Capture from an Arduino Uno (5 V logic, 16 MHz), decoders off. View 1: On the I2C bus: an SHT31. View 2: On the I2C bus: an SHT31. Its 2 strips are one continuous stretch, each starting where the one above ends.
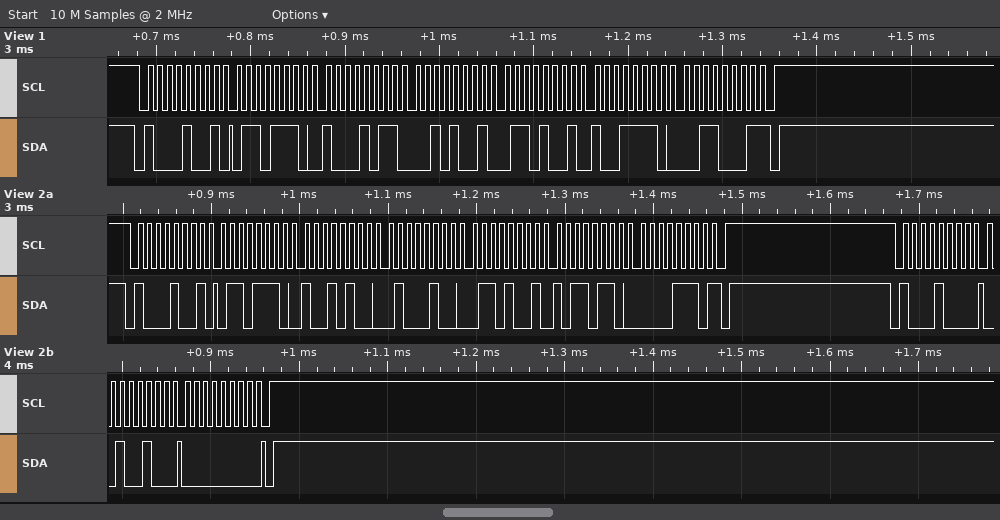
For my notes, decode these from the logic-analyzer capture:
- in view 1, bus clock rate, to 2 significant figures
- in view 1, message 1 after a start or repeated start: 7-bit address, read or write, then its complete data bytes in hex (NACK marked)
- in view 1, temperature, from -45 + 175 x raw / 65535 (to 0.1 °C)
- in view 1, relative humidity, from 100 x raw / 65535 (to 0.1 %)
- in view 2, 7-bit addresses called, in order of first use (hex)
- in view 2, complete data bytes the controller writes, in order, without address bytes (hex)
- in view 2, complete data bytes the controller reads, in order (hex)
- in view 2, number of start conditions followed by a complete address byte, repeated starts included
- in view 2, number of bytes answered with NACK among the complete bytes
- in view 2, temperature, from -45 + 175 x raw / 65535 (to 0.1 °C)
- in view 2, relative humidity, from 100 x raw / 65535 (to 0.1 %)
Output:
100 kHz
0x44 read: 6E 8B 29 69 9E 31 NACK
30.6 °C
41.3 %
0x44
24 00
6E 94 44 69 B6 0E
2
1
30.6 °C
41.3 %
